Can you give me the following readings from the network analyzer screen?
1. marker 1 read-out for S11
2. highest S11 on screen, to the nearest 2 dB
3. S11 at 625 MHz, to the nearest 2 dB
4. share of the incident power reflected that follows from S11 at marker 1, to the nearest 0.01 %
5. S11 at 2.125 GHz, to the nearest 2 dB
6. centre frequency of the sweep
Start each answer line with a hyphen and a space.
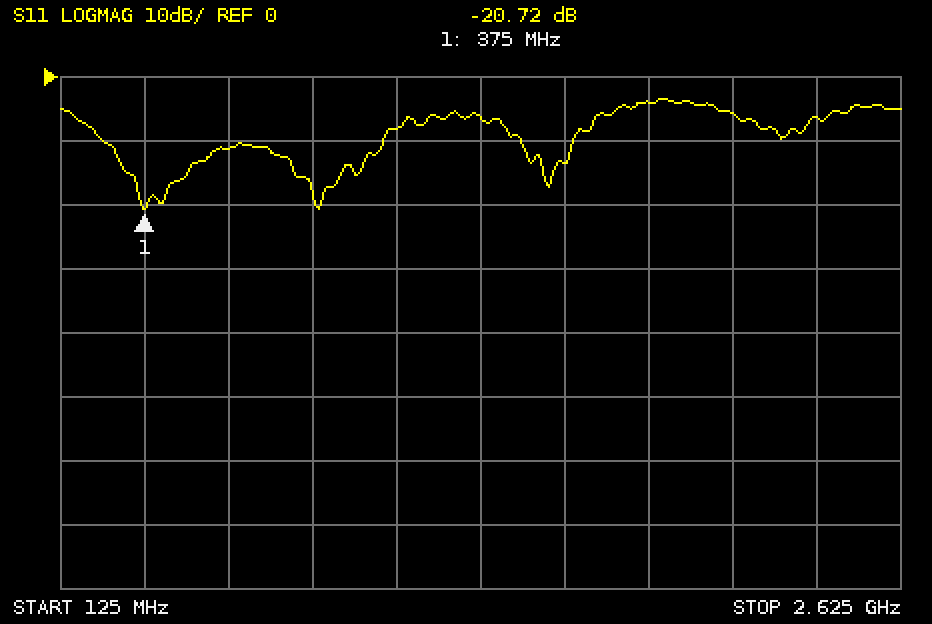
- -20.72 dB
- -4 dB
- -12 dB
- 0.85 %
- -6 dB
- 1.375 GHz
